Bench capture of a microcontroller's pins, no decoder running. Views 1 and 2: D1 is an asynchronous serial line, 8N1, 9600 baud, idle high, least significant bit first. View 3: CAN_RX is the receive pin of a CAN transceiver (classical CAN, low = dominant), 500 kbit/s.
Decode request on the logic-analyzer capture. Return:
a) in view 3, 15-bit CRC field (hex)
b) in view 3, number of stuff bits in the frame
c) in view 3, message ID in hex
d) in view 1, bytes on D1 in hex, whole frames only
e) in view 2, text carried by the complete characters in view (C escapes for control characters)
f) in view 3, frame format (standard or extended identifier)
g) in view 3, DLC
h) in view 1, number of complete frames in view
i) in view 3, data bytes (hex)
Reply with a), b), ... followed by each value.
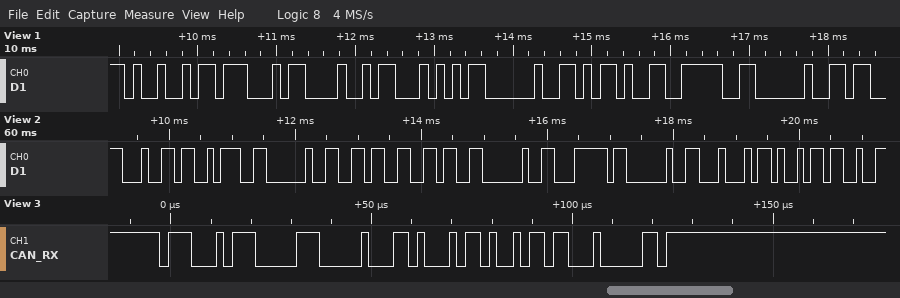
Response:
a) 0x3620
b) 3
c) 0x717
d) 49 47 48 54 20 2D 3E 20
e) "d: 66 | Di"
f) standard
g) 3
h) 8
i) 00 D1 69
